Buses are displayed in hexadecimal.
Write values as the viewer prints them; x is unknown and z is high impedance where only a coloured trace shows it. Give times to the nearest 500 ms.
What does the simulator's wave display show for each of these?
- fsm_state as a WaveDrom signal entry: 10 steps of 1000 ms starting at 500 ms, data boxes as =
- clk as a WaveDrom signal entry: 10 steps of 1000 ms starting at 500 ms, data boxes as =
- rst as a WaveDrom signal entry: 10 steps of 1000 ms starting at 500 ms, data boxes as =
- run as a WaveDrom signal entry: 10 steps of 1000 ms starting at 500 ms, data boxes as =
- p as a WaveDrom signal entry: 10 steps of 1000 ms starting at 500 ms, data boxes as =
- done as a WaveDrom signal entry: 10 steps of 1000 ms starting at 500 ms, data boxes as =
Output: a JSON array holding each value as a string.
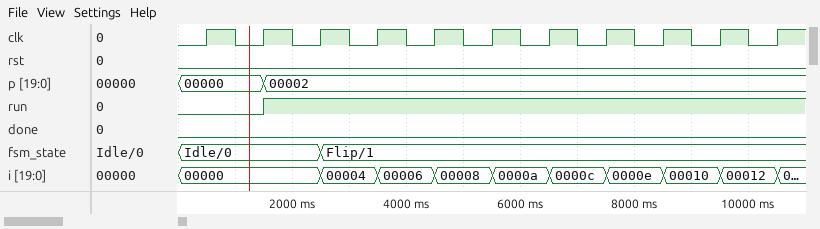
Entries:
["{name: 'fsm_state', wave: '=.=.......', data: 'Idle/0 Flip/1'}", "{name: 'clk', wave: 'p.........'}", "{name: 'rst', wave: '0.........'}", "{name: 'run', wave: '01........'}", "{name: 'p', wave: '==........', data: '00000 00002'}", "{name: 'done', wave: '0.........'}"]
